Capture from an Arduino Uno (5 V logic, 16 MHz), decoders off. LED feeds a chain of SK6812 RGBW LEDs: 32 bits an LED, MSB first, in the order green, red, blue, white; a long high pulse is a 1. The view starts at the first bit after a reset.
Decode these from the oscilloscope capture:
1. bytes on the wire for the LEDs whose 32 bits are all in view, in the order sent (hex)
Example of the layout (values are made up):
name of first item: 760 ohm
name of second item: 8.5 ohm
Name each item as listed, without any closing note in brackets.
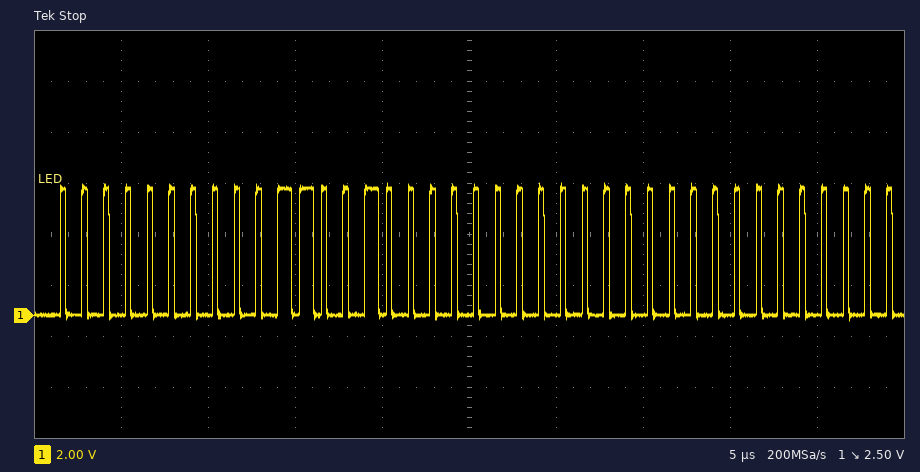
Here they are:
bytes on the wire for the LEDs whose 32 bits are all in view, in the order sent: 00 32 00 00
